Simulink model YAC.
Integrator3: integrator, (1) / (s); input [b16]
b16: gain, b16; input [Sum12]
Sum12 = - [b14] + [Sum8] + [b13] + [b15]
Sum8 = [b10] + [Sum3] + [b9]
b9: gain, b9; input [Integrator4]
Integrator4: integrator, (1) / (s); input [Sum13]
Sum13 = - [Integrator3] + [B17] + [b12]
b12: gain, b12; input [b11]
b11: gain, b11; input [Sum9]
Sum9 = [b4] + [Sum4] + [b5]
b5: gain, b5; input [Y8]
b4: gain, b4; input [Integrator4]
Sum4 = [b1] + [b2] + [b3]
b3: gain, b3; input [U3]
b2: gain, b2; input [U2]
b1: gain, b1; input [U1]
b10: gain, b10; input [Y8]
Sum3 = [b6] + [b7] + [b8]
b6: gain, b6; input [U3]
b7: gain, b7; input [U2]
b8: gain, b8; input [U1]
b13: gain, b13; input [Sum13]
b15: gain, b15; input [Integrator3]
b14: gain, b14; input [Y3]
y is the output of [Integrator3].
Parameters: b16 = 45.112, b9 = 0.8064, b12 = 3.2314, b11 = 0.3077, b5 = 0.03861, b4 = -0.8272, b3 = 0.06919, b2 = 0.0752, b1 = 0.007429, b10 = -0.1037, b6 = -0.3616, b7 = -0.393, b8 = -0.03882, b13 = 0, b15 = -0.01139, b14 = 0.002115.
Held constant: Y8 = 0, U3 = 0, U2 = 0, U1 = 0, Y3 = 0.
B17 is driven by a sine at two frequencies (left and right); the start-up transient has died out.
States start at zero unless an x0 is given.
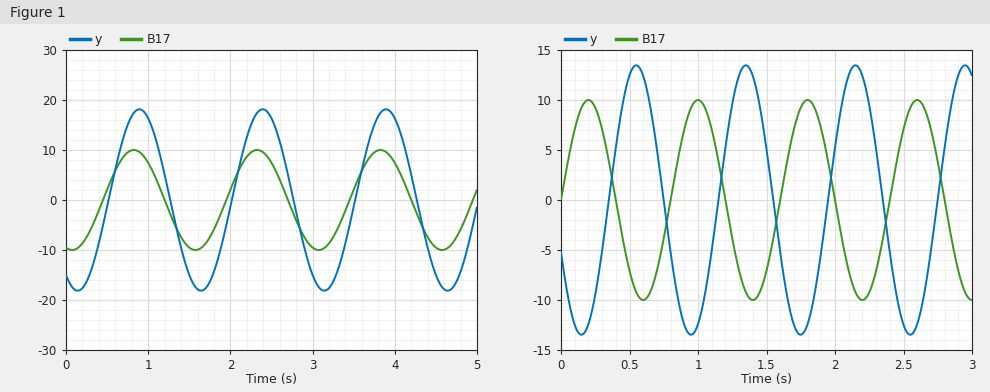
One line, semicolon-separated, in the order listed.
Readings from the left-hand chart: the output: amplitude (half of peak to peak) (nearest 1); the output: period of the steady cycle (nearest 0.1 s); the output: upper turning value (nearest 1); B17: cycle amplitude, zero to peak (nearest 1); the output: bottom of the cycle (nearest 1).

18; 1.5 s; 18; 10; -18
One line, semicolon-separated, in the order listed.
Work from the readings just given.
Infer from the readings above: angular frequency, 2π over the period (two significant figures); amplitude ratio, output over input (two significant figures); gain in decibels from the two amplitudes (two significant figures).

4.2 rad/s; 1.8; 5.1 dB
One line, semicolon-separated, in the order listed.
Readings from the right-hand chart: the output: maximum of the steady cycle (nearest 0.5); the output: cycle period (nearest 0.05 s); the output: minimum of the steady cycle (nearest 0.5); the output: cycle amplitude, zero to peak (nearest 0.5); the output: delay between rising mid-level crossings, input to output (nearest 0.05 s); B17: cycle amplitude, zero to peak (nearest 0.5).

13.5; 0.80 s; -13.5; 13.5; 0.35 s; 10.0
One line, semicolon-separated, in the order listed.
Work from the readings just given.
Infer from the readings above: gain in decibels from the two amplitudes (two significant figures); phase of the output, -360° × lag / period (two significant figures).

2.6 dB; -160°
